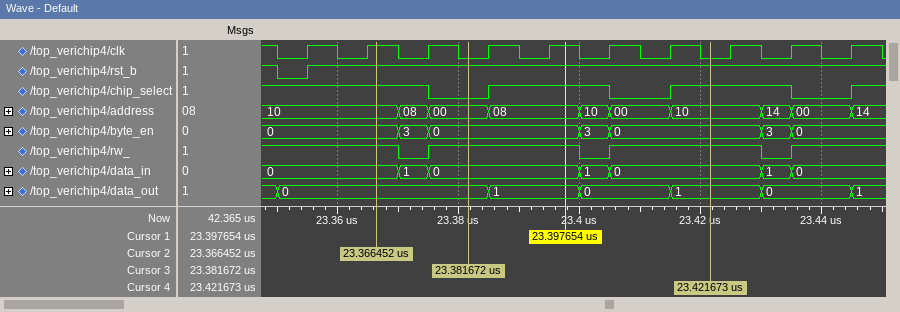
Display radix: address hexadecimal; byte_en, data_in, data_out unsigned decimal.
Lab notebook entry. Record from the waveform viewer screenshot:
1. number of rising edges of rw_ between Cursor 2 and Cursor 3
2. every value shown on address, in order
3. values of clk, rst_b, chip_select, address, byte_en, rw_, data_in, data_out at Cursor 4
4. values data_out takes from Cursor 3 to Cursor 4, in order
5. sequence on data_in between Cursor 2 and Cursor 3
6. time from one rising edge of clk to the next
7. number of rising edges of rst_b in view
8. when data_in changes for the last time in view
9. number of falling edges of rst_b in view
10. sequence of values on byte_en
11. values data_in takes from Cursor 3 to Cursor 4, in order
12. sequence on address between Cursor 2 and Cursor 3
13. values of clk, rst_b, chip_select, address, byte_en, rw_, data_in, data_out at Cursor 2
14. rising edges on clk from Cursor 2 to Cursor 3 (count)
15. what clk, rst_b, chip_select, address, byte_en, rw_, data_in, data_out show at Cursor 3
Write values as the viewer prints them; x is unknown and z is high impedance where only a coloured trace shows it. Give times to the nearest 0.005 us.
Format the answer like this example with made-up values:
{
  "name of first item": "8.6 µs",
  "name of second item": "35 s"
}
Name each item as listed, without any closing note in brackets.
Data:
{
  "number of rising edges of rw_ between Cursor 2 and Cursor 3": "1",
  "every value shown on address, in order": "10, 08, 00, 08, 10, 00, 10, 14, 00, 14",
  "values of clk, rst_b, chip_select, address, byte_en, rw_, data_in, data_out at Cursor 4": "clk=0, rst_b=1, chip_select=1, address=10, byte_en=0, rw_=1, data_in=0, data_out=1",
  "values data_out takes from Cursor 3 to Cursor 4, in order": "0, 1, 0, 1",
  "sequence on data_in between Cursor 2 and Cursor 3": "0, 1, 0",
  "time from one rising edge of clk to the next": "0.01 us",
  "number of rising edges of rst_b in view": "1",
  "when data_in changes for the last time in view": "23.435 us",
  "number of falling edges of rst_b in view": "1",
  "sequence of values on byte_en": "0, 3, 0, 3, 0, 3, 0",
  "values data_in takes from Cursor 3 to Cursor 4, in order": "0, 1, 0",
  "sequence on address between Cursor 2 and Cursor 3": "10, 08, 00",
  "values of clk, rst_b, chip_select, address, byte_en, rw_, data_in, data_out at Cursor 2": "clk=1, rst_b=1, chip_select=1, address=10, byte_en=0, rw_=1, data_in=0, data_out=0",
  "rising edges on clk from Cursor 2 to Cursor 3": "1",
  "what clk, rst_b, chip_select, address, byte_en, rw_, data_in, data_out show at Cursor 3": "clk=0, rst_b=1, chip_select=0, address=00, byte_en=0, rw_=1, data_in=0, data_out=0"
}
